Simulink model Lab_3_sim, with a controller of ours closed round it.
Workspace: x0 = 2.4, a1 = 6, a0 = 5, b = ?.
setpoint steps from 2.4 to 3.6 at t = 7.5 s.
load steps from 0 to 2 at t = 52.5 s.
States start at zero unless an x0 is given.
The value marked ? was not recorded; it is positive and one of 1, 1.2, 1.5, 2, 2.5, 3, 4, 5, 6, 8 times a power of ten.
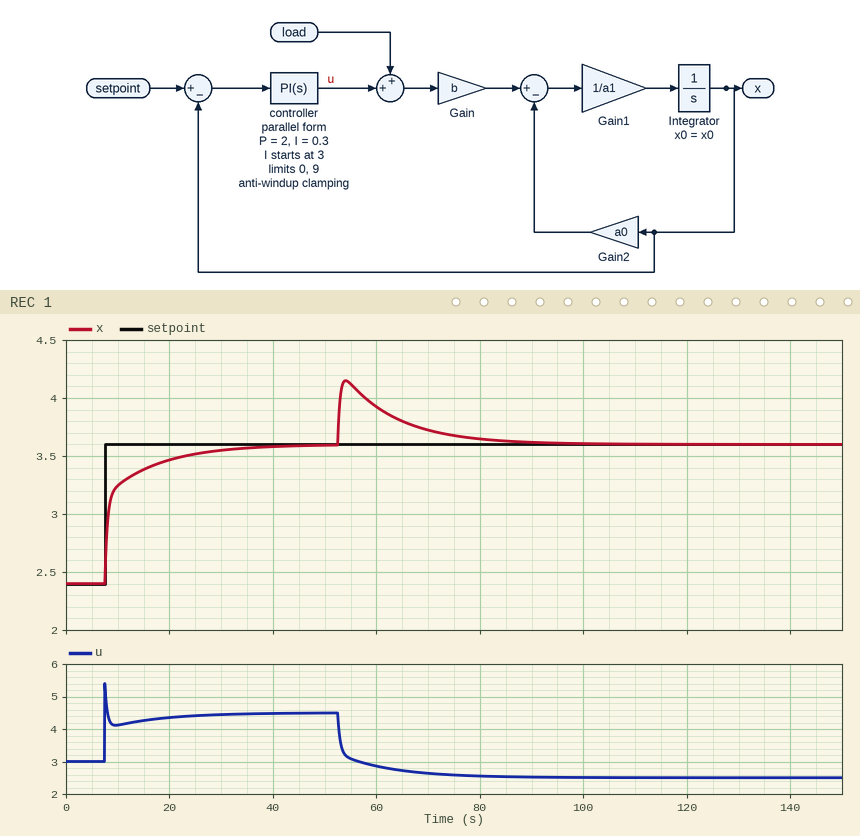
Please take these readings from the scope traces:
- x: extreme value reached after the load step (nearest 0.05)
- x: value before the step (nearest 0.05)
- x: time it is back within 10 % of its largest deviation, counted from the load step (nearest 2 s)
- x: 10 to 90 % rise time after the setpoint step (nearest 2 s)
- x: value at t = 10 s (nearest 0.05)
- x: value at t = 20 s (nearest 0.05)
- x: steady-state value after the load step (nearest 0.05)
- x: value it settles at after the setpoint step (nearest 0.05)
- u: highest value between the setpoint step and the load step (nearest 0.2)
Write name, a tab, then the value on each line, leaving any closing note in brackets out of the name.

x: extreme value reached after the load step	4.15
x: value before the step	2.40
x: time it is back within 10 % of its largest deviation, counted from the load step	26 s
x: 10 to 90 % rise time after the setpoint step	14 s
x: value at t = 10 s	3.25
x: value at t = 20 s	3.45
x: steady-state value after the load step	3.60
x: value it settles at after the setpoint step	3.60
u: highest value between the setpoint step and the load step	5.4
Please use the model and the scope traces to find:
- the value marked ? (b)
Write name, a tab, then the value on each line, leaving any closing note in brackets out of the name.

the value marked ?	4
